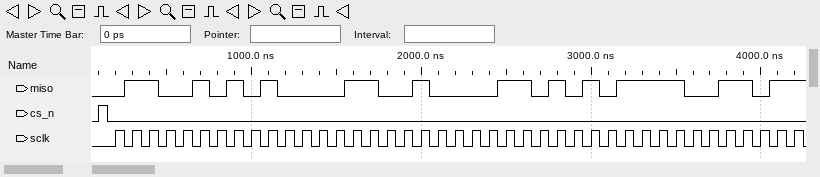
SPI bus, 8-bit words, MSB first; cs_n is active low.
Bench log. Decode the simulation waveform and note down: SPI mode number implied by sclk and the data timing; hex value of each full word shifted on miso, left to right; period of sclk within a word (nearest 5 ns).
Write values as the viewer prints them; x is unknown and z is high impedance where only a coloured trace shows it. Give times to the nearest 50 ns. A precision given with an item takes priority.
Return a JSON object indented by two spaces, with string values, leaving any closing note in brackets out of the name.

{
  "SPI mode number implied by sclk and the data timing": "0",
  "hex value of each full word shifted on miso, left to right": "65, 43, 21, AB, CD",
  "period of sclk within a word": "100 ns"
}
